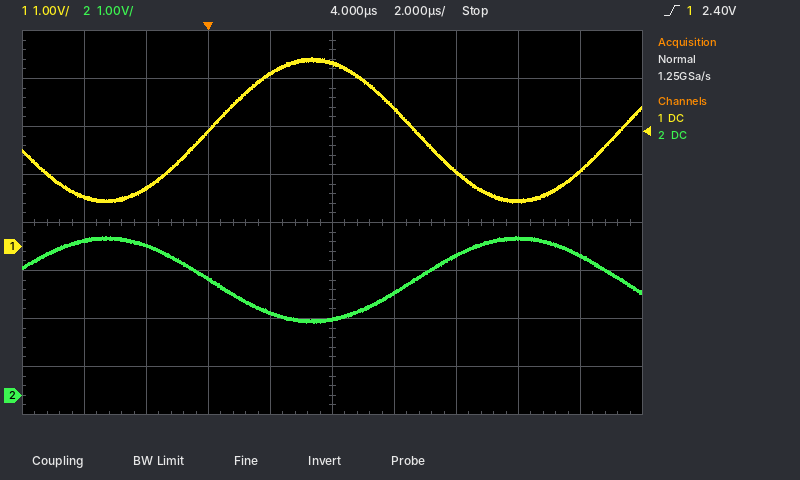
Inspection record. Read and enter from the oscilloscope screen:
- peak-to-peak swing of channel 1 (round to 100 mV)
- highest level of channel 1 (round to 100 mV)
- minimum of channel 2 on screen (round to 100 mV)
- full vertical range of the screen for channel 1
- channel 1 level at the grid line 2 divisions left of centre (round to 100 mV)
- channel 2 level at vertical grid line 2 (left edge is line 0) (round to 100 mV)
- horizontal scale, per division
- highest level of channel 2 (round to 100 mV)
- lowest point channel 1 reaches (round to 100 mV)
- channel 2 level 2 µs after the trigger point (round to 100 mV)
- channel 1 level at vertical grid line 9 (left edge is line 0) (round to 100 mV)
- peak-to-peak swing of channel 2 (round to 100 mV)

3.0 V
3.9 V
1.5 V
8 V
2.4 V
3.1 V
2 µs
3.3 V
900 mV
1.7 V
1.6 V
1.8 V
